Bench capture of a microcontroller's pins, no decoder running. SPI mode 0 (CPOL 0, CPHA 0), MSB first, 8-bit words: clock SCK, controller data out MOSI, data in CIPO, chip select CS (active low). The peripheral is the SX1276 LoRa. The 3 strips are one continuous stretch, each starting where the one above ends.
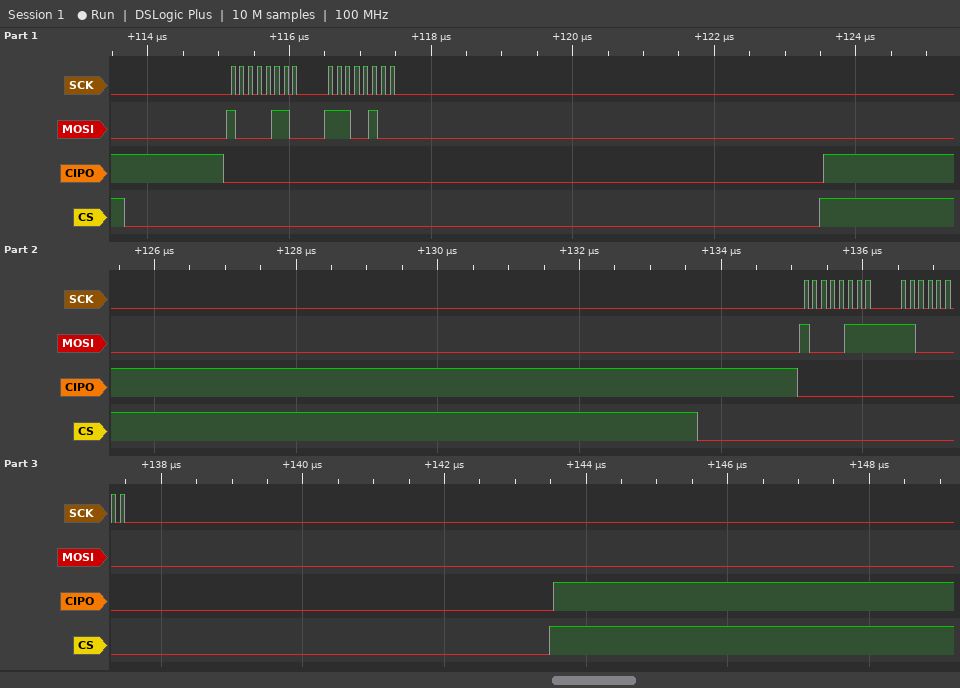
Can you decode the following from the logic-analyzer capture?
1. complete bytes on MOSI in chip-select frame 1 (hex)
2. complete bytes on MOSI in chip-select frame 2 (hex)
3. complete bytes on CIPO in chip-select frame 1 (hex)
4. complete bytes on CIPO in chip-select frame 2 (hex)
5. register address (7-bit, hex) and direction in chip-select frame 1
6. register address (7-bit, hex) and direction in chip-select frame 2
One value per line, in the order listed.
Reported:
86 E4
87 C0
00 00
00 00
0x06 write
0x07 write
